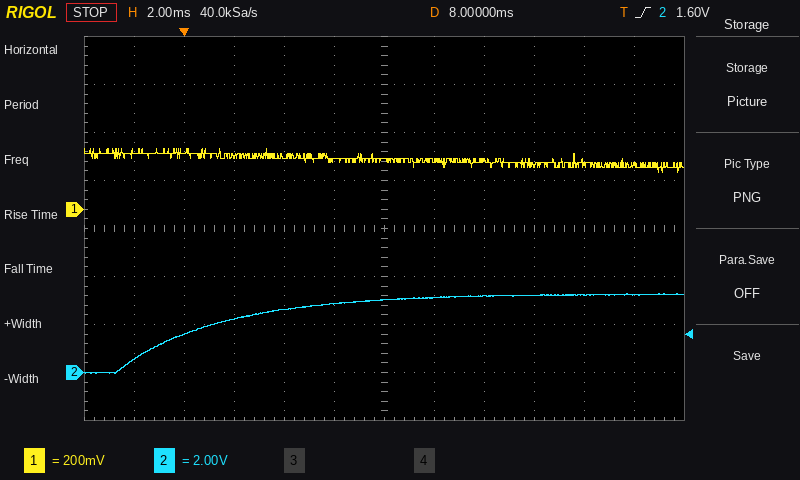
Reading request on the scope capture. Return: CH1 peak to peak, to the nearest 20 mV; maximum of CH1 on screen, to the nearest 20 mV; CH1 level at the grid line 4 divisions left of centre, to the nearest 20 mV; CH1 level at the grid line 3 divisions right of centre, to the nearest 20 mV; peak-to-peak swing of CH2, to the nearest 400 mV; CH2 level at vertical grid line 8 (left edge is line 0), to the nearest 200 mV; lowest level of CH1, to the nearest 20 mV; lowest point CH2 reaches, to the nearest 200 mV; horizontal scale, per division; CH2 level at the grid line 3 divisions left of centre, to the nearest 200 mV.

100 mV
260 mV
240 mV
180 mV
3.2 V
3.2 V
160 mV
0.0 V
2 ms
2.2 V
